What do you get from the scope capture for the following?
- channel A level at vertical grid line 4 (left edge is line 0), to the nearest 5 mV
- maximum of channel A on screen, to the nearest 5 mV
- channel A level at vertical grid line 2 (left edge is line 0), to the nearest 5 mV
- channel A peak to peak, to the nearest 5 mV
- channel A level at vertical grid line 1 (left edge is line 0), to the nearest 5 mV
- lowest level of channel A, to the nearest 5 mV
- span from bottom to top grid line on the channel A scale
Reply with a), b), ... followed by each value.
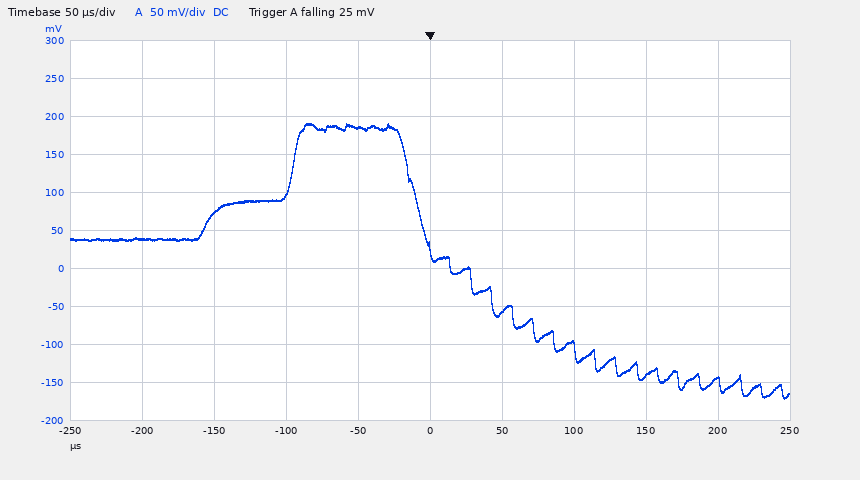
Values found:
a) 185 mV
b) 190 mV
c) 75 mV
d) 360 mV
e) 40 mV
f) -170 mV
g) 500 mV
